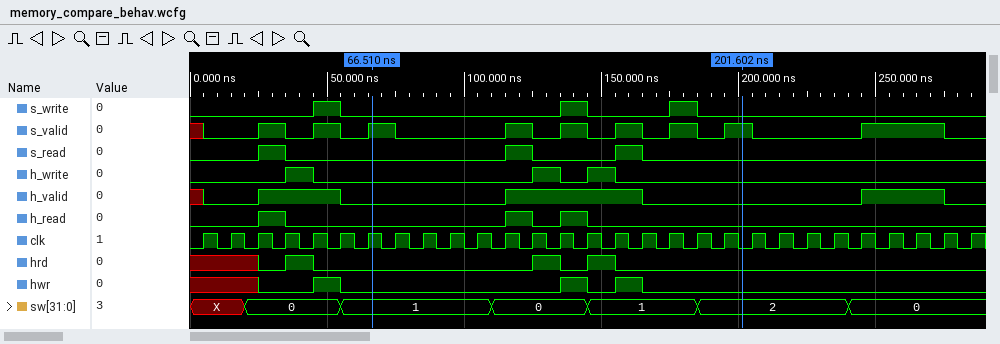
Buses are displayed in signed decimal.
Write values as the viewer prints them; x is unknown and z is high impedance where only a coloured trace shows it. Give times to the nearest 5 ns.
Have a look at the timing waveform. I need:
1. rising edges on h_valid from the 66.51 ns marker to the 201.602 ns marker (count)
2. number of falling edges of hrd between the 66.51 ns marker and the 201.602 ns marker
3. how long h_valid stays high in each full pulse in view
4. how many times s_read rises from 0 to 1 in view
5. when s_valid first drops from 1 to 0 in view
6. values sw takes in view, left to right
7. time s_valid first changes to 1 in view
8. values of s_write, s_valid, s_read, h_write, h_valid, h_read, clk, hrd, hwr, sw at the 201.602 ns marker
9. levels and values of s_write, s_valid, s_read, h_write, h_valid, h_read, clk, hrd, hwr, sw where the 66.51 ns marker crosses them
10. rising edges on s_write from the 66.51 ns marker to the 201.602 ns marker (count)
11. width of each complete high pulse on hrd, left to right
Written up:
1
2
30 ns, 50 ns, 30 ns
3
35 ns
X, 0, 1, 0, 1, 2, 0
25 ns
s_write=0, s_valid=1, s_read=0, h_write=0, h_valid=0, h_read=0, clk=0, hrd=0, hwr=0, sw=2
s_write=0, s_valid=1, s_read=0, h_write=0, h_valid=0, h_read=0, clk=1, hrd=0, hwr=0, sw=1
2
10 ns, 10 ns, 10 ns
